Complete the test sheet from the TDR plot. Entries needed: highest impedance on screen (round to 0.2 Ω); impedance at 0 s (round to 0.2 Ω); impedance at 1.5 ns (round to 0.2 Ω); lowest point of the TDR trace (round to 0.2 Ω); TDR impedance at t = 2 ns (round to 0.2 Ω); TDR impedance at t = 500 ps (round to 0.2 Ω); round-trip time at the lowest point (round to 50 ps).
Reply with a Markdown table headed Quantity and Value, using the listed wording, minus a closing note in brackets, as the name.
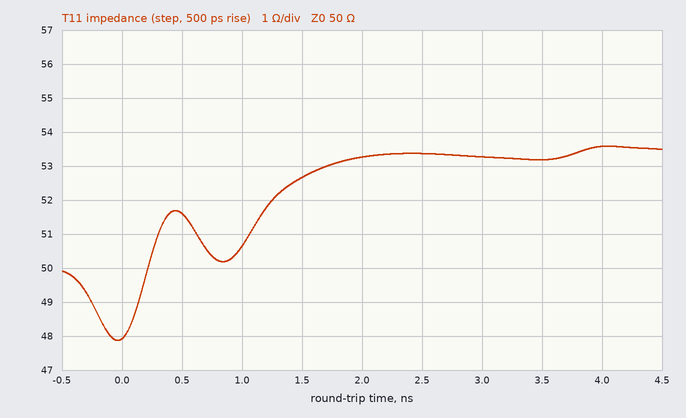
| Quantity | Value |
|---|---|
| highest impedance on screen | 53.6 Ω |
| impedance at 0 s | 48.0 Ω |
| impedance at 1.5 ns | 52.6 Ω |
| lowest point of the TDR trace | 47.8 Ω |
| TDR impedance at t = 2 ns | 53.2 Ω |
| TDR impedance at t = 500 ps | 51.6 Ω |
| round-trip time at the lowest point | -50 ps |
